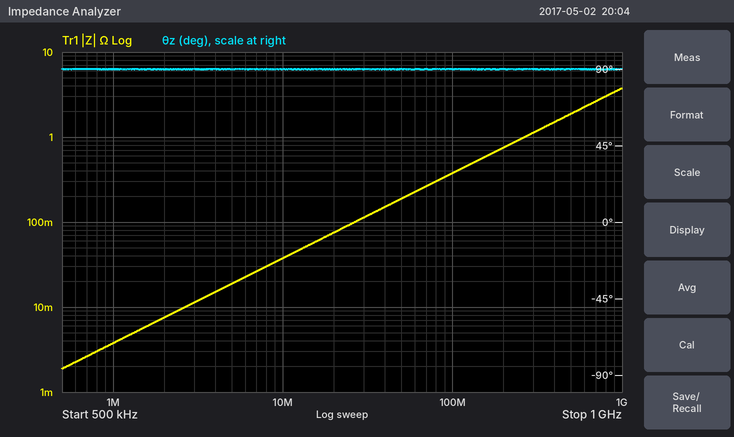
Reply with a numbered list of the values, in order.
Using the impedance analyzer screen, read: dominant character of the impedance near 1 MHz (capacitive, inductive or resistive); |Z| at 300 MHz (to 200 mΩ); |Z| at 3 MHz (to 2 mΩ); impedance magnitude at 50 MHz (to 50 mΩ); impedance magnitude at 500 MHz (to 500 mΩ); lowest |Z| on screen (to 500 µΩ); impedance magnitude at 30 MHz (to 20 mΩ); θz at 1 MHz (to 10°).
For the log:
1. inductive
2. 1.2 Ω
3. 12 mΩ
4. 200 mΩ
5. 2.0 Ω
6. 2.0 mΩ
7. 120 mΩ
8. 90°
